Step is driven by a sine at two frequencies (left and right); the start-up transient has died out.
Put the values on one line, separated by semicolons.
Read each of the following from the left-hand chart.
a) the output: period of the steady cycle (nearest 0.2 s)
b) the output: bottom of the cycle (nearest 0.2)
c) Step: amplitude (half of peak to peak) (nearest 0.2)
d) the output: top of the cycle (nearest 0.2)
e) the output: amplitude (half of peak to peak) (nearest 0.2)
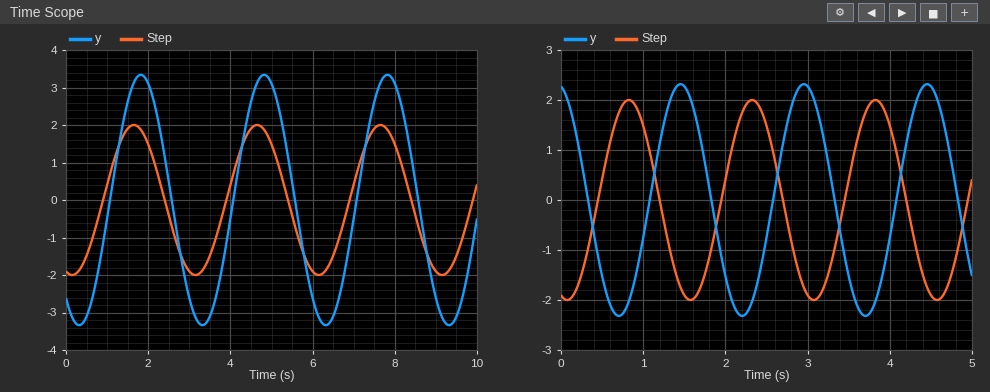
3.0 s; -3.4; 2.0; 3.4; 3.4
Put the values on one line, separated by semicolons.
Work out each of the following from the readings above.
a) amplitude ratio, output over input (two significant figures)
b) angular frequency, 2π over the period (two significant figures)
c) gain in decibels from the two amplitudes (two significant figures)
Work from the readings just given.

1.7; 2.1 rad/s; 4.6 dB
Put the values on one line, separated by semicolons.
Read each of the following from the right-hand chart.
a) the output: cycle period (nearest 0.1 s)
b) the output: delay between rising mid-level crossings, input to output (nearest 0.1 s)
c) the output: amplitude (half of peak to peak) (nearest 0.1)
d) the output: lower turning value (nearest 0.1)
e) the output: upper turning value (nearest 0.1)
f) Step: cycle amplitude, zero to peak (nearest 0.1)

1.5 s; 0.6 s; 2.3; -2.3; 2.3; 2.0
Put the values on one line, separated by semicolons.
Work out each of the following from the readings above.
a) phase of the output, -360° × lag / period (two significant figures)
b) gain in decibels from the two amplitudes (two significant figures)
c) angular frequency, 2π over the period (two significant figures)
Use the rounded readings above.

-140°; 1.2 dB; 4.2 rad/s
